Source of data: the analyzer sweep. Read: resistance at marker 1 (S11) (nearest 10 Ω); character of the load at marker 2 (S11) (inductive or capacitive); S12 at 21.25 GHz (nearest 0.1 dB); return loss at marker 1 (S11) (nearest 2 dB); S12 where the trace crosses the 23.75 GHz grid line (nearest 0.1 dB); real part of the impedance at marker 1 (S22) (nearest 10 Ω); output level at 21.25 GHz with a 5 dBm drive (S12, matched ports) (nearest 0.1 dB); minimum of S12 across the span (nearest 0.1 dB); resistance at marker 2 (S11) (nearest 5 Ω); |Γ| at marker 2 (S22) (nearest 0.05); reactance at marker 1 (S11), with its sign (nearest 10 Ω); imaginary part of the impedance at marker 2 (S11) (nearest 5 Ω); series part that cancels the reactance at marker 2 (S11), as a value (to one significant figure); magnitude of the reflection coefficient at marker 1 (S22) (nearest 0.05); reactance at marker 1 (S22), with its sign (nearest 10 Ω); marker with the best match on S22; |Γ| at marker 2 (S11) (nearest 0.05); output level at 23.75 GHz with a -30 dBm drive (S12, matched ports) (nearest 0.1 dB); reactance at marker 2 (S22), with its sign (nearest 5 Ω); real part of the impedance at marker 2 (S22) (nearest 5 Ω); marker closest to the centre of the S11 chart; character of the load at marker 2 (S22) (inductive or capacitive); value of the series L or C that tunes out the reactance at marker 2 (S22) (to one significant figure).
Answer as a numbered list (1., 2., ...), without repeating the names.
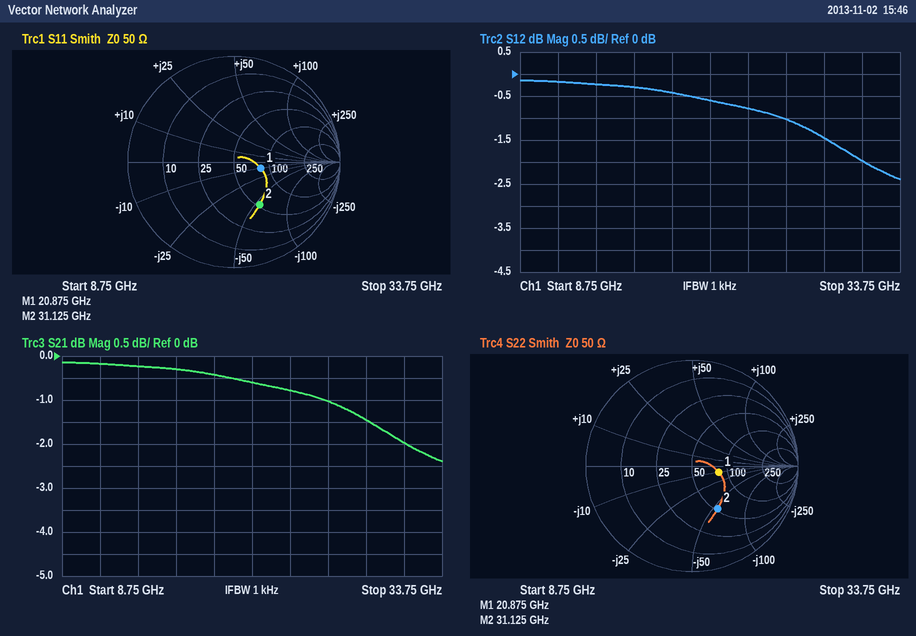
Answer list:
1. 80 Ω
2. capacitive
3. -0.6 dB
4. 12 dB
5. -0.8 dB
6. 80 Ω
7. 4.4 dBm
8. -2.4 dB
9. 55 Ω
10. 0.45
11. -10 Ω
12. -55 Ω
13. 300 pH
14. 0.25
15. -10 Ω
16. marker 1
17. 0.45
18. -30.8 dBm
19. -55 Ω
20. 55 Ω
21. marker 1
22. capacitive
23. 300 pH
